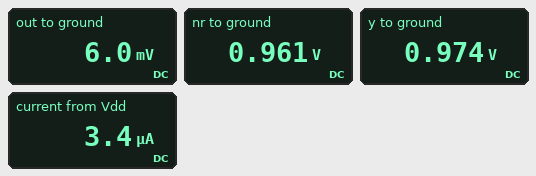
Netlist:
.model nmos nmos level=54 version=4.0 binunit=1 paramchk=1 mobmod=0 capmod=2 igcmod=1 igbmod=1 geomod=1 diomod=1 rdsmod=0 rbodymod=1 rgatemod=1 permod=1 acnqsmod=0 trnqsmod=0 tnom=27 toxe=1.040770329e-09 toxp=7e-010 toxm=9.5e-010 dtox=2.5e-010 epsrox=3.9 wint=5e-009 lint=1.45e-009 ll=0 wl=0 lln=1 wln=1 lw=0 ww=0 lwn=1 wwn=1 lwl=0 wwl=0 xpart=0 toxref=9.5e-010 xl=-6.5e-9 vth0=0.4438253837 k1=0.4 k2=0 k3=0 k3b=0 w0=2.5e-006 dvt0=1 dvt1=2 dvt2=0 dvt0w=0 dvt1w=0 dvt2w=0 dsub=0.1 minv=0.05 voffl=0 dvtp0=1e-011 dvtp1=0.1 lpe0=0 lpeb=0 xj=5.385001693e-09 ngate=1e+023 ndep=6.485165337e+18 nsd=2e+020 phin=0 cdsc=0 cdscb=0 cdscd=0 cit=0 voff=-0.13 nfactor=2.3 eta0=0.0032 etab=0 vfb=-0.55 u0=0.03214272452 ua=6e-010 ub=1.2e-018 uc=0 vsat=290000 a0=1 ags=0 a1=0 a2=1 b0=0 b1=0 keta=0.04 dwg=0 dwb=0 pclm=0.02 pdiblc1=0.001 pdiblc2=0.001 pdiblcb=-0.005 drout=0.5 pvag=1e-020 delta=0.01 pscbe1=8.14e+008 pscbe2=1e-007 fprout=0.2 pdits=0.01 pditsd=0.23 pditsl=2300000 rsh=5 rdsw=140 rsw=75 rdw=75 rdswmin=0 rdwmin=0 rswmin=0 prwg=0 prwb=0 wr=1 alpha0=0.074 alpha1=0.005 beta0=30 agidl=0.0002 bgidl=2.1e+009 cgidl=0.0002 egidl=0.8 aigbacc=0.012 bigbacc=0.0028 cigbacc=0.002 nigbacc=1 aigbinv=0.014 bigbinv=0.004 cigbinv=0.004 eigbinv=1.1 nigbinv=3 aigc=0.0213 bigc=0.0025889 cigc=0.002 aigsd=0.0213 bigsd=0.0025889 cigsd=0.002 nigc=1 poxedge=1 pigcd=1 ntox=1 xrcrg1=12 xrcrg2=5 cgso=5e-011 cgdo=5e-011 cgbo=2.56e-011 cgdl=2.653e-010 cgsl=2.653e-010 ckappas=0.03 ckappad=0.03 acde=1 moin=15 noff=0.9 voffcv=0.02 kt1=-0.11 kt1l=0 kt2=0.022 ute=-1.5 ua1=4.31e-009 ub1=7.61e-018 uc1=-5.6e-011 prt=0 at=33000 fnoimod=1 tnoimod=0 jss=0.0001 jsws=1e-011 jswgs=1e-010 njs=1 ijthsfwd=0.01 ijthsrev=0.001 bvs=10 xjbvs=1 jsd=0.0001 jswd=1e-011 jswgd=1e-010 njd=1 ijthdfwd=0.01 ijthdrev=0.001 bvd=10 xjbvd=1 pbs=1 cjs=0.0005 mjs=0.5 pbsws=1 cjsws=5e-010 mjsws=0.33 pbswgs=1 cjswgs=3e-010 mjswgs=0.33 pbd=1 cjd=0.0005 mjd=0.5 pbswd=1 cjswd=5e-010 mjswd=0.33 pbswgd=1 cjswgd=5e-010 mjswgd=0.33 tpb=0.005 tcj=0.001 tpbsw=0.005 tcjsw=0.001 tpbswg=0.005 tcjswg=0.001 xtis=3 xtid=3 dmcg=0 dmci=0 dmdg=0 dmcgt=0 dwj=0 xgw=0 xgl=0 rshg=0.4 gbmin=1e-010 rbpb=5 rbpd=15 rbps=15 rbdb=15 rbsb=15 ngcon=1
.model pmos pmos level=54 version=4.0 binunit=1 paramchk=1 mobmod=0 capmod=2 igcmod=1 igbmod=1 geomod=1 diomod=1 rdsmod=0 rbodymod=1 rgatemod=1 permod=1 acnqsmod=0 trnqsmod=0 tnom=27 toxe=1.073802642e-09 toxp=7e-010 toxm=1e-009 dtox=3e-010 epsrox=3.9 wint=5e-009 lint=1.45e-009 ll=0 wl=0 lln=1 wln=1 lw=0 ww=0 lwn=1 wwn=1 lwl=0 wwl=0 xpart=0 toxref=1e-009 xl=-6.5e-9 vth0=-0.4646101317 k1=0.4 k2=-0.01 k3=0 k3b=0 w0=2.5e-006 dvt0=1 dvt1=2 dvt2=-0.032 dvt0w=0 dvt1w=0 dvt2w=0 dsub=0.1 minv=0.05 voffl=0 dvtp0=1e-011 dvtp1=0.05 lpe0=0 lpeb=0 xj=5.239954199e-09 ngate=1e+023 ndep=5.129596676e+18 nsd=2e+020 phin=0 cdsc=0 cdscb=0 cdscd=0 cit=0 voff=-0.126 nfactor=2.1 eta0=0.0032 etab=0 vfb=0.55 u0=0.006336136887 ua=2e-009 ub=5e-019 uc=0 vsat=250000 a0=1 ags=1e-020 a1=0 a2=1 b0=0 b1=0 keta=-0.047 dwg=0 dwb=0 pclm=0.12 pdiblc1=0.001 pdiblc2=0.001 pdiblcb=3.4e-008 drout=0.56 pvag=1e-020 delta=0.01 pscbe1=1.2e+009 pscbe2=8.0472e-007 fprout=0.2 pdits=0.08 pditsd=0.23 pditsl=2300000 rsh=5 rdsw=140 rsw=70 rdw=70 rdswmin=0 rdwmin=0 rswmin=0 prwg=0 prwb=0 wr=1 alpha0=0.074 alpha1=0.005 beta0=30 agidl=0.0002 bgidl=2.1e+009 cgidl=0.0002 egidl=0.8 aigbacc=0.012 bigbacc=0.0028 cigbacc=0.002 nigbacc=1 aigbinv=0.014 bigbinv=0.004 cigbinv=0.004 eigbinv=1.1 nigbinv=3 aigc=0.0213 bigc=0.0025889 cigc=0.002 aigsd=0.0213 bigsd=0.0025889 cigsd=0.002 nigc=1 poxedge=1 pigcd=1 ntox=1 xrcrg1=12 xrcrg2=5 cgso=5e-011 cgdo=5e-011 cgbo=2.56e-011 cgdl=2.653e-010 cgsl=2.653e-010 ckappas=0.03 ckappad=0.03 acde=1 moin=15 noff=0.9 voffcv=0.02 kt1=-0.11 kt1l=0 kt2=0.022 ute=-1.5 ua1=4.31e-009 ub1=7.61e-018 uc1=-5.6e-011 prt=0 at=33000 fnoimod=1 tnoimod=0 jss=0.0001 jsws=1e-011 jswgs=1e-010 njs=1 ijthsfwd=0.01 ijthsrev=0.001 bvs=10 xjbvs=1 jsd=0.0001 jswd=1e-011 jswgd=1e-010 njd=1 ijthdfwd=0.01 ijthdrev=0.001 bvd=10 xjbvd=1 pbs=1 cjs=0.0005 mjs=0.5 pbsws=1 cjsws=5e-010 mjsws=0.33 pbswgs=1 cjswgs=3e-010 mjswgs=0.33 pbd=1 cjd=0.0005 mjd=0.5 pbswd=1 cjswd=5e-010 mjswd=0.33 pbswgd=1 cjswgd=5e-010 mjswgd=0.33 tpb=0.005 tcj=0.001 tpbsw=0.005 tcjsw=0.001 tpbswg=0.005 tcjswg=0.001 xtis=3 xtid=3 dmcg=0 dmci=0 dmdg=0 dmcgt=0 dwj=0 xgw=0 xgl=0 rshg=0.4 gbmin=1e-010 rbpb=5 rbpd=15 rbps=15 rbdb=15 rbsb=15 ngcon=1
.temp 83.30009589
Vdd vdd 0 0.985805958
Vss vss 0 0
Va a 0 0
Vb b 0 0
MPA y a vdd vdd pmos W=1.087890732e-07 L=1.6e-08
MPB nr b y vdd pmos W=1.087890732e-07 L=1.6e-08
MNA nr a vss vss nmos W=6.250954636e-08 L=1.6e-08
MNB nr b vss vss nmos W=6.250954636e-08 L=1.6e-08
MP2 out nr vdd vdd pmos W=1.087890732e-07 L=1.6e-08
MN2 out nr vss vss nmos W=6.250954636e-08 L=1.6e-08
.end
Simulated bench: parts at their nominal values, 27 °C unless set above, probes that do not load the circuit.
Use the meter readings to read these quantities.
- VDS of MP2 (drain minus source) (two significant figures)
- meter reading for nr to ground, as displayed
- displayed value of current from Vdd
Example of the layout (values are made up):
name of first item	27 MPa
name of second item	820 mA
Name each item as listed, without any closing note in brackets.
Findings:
VDS of MP2 (drain minus source)	-980 mV
meter reading for nr to ground, as displayed	0.961 V
displayed value of current from Vdd	3.4 µA
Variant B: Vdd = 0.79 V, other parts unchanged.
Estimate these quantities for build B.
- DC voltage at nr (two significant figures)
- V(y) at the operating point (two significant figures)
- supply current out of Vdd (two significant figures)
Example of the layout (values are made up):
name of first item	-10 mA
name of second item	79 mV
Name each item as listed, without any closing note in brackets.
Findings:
DC voltage at nr	780 mV
V(y) at the operating point	790 mV
supply current out of Vdd	630 nA
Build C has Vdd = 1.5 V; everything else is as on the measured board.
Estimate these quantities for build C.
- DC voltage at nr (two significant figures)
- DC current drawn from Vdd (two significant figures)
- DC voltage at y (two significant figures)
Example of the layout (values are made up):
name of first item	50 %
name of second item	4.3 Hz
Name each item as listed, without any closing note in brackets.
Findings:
DC voltage at nr	1.3 V
DC current drawn from Vdd	91 µA
DC voltage at y	1.4 V
